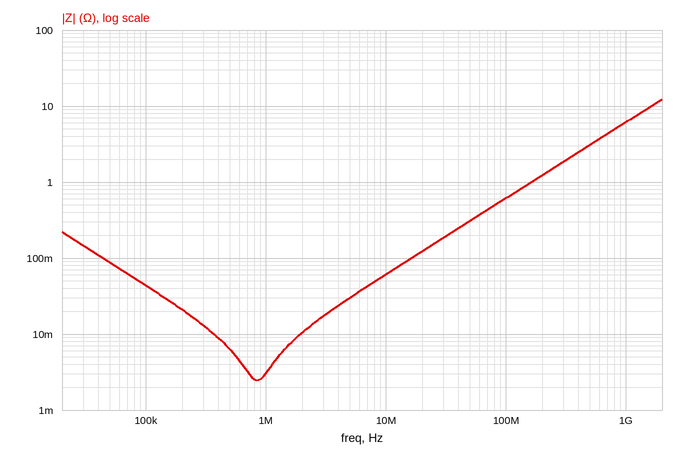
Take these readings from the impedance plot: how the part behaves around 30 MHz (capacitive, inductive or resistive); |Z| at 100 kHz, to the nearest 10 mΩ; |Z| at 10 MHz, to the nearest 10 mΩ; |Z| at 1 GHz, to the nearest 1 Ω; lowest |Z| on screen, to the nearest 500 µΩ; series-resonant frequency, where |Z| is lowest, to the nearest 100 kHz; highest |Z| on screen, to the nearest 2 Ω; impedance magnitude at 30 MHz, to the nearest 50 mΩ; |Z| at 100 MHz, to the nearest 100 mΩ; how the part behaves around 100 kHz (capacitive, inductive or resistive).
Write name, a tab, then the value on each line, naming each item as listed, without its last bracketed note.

how the part behaves around 30 MHz	inductive
|Z| at 100 kHz, to the nearest 10 mΩ	40 mΩ
|Z| at 10 MHz, to the nearest 10 mΩ	60 mΩ
|Z| at 1 GHz, to the nearest 1 Ω	6 Ω
lowest |Z| on screen, to the nearest 500 µΩ	2.5 mΩ
series-resonant frequency, where |Z| is lowest, to the nearest 100 kHz	800 kHz
highest |Z| on screen, to the nearest 2 Ω	12 Ω
impedance magnitude at 30 MHz, to the nearest 50 mΩ	200 mΩ
|Z| at 100 MHz, to the nearest 100 mΩ	600 mΩ
how the part behaves around 100 kHz	capacitive
